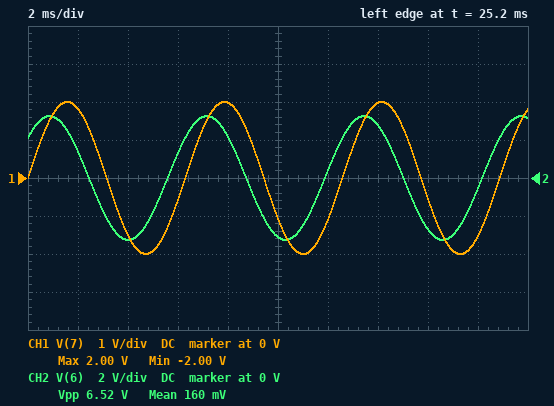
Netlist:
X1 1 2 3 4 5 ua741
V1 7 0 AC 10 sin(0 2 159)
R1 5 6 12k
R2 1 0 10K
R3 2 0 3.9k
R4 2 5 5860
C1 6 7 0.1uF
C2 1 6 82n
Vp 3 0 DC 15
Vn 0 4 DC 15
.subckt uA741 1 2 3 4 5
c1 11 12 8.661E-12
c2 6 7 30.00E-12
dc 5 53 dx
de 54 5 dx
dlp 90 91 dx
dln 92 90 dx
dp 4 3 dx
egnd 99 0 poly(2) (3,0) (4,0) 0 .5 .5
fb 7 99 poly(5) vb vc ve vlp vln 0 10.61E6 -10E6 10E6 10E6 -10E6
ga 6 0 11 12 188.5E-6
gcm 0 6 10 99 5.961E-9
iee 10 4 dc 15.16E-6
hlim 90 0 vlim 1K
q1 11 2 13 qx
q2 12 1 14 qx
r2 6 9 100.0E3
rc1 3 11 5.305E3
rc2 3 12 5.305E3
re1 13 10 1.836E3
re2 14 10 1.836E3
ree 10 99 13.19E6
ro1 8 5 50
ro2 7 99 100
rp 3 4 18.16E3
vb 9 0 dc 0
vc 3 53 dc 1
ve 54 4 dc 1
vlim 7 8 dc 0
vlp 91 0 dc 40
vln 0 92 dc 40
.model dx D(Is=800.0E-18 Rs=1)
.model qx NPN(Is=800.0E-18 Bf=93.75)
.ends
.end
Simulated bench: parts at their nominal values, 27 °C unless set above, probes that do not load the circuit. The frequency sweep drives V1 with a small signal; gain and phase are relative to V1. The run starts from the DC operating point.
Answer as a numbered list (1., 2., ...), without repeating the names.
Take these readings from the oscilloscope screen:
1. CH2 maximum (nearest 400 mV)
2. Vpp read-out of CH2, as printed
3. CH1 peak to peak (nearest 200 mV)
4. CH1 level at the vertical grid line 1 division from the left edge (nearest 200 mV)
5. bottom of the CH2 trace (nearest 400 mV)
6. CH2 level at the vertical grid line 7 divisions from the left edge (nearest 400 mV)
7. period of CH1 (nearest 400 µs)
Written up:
1. 3.2 V
2. 6.52 V
3. 4.0 V
4. 1.8 V
5. -3.2 V
6. 2.8 V
7. 6.4 ms
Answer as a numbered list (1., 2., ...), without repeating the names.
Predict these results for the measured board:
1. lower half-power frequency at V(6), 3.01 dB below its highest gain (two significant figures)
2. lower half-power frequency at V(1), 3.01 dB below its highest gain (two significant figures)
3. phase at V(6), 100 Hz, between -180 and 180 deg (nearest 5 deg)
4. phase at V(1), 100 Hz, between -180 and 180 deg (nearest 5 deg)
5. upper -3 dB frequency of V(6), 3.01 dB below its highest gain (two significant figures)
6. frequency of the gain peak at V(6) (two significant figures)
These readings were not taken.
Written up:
1. 110 Hz
2. 140 Hz
3. 75 deg
4. 135 deg
5. 420 Hz
6. 180 Hz
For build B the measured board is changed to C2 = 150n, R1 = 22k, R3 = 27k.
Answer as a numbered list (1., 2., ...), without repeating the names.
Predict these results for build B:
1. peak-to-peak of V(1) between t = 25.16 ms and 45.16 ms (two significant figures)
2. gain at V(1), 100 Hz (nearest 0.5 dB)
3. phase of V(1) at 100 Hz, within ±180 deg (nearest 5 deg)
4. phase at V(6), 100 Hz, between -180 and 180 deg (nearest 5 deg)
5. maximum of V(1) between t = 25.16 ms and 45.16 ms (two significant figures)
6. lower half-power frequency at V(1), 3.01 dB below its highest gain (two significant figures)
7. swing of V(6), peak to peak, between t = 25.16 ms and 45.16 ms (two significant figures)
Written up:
1. 2.3 V
2. -8.0 dB
3. 85 deg
4. 40 deg
5. 1.2 V
6. 220 Hz
7. 2.8 V
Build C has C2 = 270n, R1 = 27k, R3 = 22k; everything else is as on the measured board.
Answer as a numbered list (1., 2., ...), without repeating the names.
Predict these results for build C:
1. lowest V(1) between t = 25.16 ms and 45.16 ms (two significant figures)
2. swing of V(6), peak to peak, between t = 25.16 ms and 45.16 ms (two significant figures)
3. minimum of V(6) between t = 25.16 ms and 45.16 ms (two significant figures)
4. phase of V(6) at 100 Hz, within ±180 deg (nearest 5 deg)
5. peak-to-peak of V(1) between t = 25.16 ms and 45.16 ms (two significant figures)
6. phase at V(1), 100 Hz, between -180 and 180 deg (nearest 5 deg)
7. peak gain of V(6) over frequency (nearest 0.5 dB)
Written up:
1. -1.3 V
2. 2.8 V
3. -1.4 V
4. 40 deg
5. 2.6 V
6. 70 deg
7. 0 dB
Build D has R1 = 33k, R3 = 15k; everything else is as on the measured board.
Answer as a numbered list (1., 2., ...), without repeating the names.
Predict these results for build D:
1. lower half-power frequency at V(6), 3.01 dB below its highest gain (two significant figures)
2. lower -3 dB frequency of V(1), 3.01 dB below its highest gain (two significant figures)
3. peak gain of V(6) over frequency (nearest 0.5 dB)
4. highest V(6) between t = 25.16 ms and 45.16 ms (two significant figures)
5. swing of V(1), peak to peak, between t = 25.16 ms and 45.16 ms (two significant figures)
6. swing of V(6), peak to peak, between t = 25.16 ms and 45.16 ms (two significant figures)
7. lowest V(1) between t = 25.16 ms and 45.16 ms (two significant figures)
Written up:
1. 150 Hz
2. 310 Hz
3. 0 dB
4. 1.4 V
5. 1.8 V
6. 2.9 V
7. -910 mV
